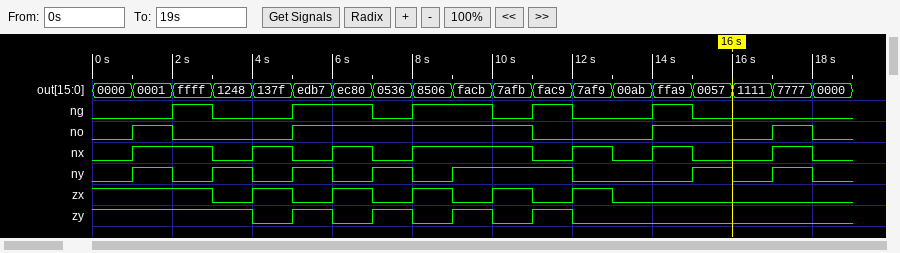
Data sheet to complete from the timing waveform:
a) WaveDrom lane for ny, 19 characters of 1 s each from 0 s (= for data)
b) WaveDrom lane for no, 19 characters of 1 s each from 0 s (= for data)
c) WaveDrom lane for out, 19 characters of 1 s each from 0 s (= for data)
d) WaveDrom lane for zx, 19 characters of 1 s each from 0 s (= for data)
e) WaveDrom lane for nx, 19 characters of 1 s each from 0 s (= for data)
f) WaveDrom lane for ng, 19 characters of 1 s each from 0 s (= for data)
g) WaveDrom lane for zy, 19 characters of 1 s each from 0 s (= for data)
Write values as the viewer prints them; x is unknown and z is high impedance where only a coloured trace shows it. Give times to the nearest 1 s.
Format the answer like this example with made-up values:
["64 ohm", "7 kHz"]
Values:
["{name: 'ny', wave: '0101010101..0..1010'}", "{name: 'no', wave: '010..1.....0..1.010'}", "{name: 'out', wave: '===================', data: '0000 0001 ffff 1248 137f edb7 ec80 0536 8506 facb 7afb fac9 7af9 00ab ffa9 0057 1111 7777 0000'}", "{name: 'zx', wave: '1..01010101010.....'}", "{name: 'nx', wave: '01.010101..01010.10'}", "{name: 'ng', wave: '0.10.1.01.010.10...'}", "{name: 'zy', wave: '1...010101010......'}"]
